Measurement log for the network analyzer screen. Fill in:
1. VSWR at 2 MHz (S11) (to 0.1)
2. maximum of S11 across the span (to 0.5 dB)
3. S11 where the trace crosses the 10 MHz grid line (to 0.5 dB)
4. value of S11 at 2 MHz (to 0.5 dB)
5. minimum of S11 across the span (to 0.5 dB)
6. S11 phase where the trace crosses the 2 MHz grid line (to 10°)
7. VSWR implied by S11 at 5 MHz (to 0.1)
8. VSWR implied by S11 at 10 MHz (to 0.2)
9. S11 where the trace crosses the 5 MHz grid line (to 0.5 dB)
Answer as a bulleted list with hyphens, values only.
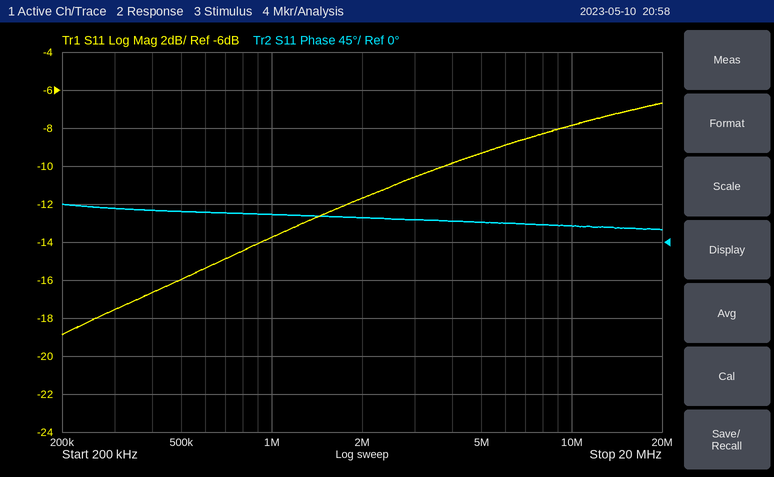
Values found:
- 1.7
- -6.5 dB
- -8.0 dB
- -11.5 dB
- -19.0 dB
- 30°
- 2.0
- 2.4
- -9.5 dB
